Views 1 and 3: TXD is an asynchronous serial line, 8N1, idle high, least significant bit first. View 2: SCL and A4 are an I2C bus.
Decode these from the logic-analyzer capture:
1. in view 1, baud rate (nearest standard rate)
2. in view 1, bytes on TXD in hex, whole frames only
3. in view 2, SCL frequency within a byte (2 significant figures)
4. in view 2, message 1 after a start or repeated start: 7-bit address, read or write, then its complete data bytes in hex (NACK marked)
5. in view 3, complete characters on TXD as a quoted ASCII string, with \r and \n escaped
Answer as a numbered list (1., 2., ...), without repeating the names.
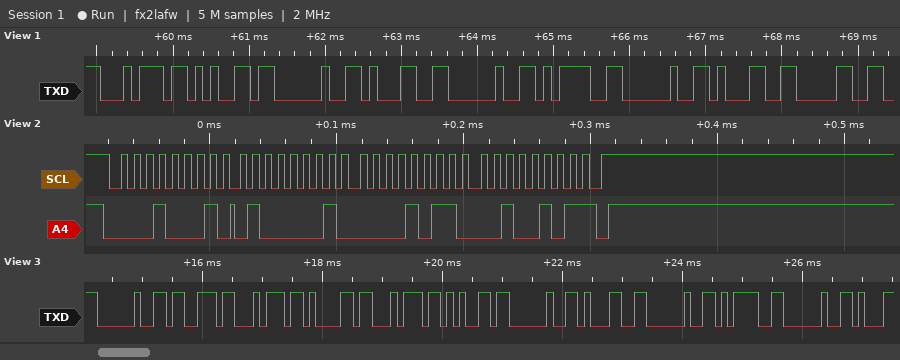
1. 9600 baud
2. 74 65 20 31 20 3D 20 31 30
3. 100 kHz
4. 0x08 read: 41 0B 25 NACK
5. " state 1 = "
